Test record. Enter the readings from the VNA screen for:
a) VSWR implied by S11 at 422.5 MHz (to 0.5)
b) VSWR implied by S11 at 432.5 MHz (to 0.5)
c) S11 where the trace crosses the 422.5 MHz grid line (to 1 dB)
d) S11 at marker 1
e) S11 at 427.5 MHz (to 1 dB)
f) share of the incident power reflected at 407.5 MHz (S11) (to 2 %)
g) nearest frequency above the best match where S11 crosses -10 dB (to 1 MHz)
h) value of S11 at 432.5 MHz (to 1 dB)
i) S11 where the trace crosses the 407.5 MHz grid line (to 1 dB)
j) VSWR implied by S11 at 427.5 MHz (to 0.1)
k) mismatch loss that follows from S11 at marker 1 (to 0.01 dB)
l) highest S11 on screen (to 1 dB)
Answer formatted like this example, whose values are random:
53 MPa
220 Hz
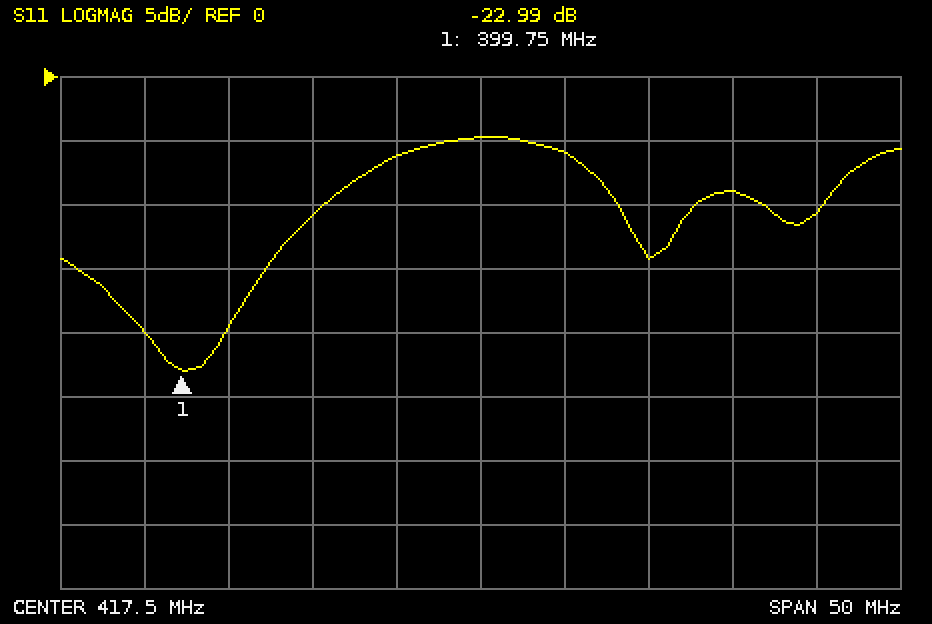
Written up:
3.0
2.0
-6 dB
-22.99 dB
-14 dB
8 %
408 MHz
-9 dB
-11 dB
1.5
0.02 dB
-5 dB
